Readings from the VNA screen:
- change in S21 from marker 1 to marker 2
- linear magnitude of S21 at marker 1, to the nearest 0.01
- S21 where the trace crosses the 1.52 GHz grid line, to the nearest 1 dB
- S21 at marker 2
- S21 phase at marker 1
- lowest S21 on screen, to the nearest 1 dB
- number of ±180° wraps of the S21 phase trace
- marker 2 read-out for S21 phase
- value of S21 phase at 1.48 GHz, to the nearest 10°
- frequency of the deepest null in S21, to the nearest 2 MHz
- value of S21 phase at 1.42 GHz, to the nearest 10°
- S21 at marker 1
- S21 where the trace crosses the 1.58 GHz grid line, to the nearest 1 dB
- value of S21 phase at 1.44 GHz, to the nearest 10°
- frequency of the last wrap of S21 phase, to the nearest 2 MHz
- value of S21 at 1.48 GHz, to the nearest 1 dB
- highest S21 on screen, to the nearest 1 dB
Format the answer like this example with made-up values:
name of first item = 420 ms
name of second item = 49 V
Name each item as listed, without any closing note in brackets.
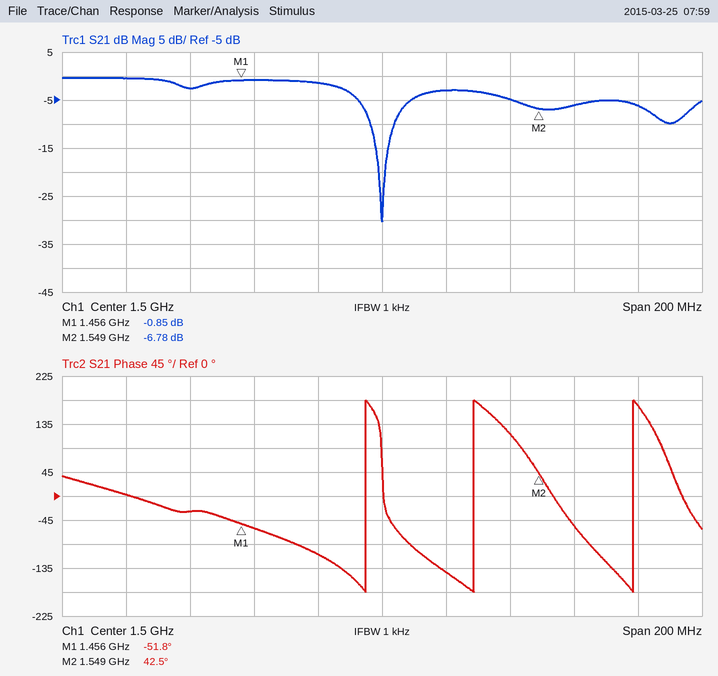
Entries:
change in S21 from marker 1 to marker 2 = -5.93 dB
linear magnitude of S21 at marker 1, to the nearest 0.01 = 0.91
S21 where the trace crosses the 1.52 GHz grid line, to the nearest 1 dB = -3 dB
S21 at marker 2 = -6.78 dB
S21 phase at marker 1 = -51.8°
lowest S21 on screen, to the nearest 1 dB = -30 dB
number of ±180° wraps of the S21 phase trace = 3
marker 2 read-out for S21 phase = 42.5°
value of S21 phase at 1.48 GHz, to the nearest 10° = -110°
frequency of the deepest null in S21, to the nearest 2 MHz = 1.500 GHz
value of S21 phase at 1.42 GHz, to the nearest 10° = 0°
S21 at marker 1 = -0.85 dB
S21 where the trace crosses the 1.58 GHz grid line, to the nearest 1 dB = -6 dB
value of S21 phase at 1.44 GHz, to the nearest 10° = -30°
frequency of the last wrap of S21 phase, to the nearest 2 MHz = 1.578 GHz
value of S21 at 1.48 GHz, to the nearest 1 dB = -1 dB
highest S21 on screen, to the nearest 1 dB = 0 dB
